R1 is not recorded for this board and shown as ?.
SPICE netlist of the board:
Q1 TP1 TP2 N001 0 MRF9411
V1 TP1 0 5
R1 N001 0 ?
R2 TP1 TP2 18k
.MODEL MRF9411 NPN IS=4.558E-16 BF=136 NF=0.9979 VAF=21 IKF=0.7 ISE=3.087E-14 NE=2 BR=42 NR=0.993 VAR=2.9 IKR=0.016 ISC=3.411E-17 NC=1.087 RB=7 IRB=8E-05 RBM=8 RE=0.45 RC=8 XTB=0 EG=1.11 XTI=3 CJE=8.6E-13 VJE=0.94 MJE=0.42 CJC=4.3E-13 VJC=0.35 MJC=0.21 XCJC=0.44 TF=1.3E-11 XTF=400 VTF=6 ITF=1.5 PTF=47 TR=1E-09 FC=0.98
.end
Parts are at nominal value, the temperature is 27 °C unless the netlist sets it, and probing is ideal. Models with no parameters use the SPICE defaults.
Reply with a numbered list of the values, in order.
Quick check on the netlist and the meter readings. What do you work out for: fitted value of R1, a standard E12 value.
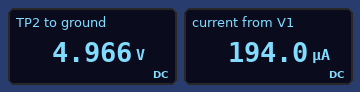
1. 22 kΩ
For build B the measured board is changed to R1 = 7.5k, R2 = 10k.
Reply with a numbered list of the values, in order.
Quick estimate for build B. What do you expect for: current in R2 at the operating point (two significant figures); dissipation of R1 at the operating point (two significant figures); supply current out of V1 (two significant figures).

1. 5.5 µA
2. 2.4 mW
3. 560 µA
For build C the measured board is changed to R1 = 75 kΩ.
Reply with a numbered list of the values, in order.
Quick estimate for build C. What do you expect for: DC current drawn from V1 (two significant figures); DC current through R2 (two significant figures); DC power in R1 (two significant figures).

1. 58 µA
2. 560 nA
3. 250 µW
